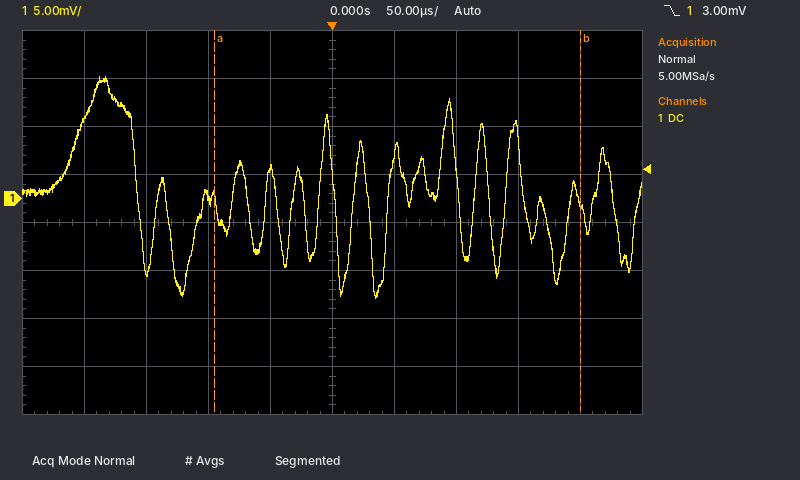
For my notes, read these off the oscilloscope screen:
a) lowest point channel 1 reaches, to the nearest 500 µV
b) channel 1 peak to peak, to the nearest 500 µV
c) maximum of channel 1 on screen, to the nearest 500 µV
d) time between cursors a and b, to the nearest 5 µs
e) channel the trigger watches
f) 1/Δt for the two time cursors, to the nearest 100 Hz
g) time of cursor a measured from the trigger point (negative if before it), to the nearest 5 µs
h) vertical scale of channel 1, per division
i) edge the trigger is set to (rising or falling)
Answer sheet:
-10.5 mV
23.0 mV
12.5 mV
295 µs
channel 1
3.4 kHz
-95 µs
5 mV
falling
